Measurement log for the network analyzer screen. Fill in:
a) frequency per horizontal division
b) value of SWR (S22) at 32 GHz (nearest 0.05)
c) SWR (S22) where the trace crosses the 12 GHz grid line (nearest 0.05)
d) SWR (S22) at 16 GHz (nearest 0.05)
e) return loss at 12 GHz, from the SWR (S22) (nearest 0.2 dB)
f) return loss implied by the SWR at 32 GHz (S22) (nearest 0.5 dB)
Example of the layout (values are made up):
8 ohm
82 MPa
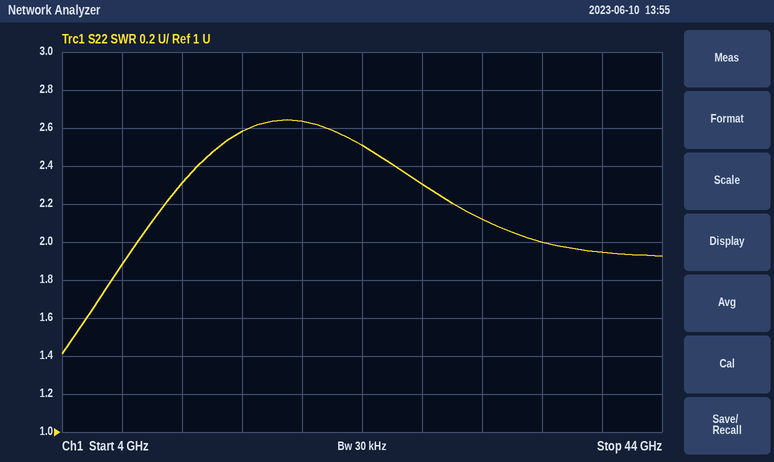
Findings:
4 GHz
2.10
2.30
2.60
8.0 dB
9.0 dB
